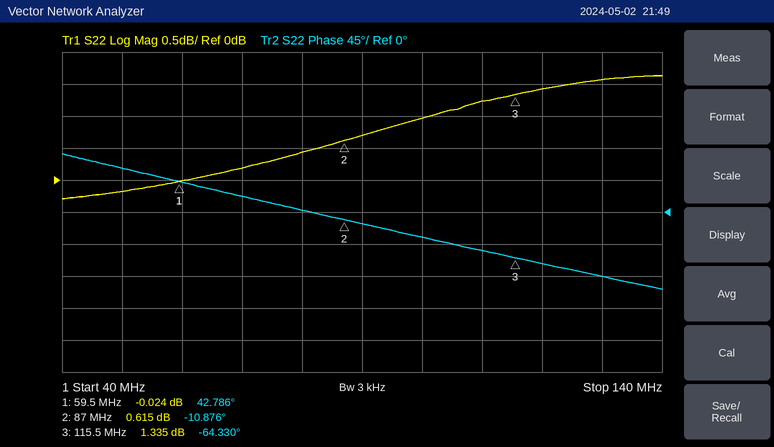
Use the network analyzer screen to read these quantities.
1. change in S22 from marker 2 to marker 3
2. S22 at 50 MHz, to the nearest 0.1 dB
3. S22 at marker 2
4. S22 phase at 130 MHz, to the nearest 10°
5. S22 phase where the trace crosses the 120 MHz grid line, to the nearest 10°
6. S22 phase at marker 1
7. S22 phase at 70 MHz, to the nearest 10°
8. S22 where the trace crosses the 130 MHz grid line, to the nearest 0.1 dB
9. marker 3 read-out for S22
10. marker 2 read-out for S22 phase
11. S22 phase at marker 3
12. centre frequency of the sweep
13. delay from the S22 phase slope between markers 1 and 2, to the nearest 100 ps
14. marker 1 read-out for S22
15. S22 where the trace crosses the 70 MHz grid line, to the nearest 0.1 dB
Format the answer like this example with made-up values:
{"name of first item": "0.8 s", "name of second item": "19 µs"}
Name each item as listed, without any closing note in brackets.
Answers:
{"change in S22 from marker 2 to marker 3": "0.720 dB", "S22 at 50 MHz, to the nearest 0.1 dB": "-0.2 dB", "S22 at marker 2": "0.615 dB", "S22 phase at 130 MHz, to the nearest 10°": "-90°", "S22 phase where the trace crosses the 120 MHz grid line, to the nearest 10°": "-70°", "S22 phase at marker 1": "42.786°", "S22 phase at 70 MHz, to the nearest 10°": "20°", "S22 where the trace crosses the 130 MHz grid line, to the nearest 0.1 dB": "1.6 dB", "marker 3 read-out for S22": "1.335 dB", "marker 2 read-out for S22 phase": "-10.876°", "S22 phase at marker 3": "-64.330°", "centre frequency of the sweep": "90 MHz", "delay from the S22 phase slope between markers 1 and 2, to the nearest 100 ps": "5.4 ns", "marker 1 read-out for S22": "-0.024 dB", "S22 where the trace crosses the 70 MHz grid line, to the nearest 0.1 dB": "0.2 dB"}
